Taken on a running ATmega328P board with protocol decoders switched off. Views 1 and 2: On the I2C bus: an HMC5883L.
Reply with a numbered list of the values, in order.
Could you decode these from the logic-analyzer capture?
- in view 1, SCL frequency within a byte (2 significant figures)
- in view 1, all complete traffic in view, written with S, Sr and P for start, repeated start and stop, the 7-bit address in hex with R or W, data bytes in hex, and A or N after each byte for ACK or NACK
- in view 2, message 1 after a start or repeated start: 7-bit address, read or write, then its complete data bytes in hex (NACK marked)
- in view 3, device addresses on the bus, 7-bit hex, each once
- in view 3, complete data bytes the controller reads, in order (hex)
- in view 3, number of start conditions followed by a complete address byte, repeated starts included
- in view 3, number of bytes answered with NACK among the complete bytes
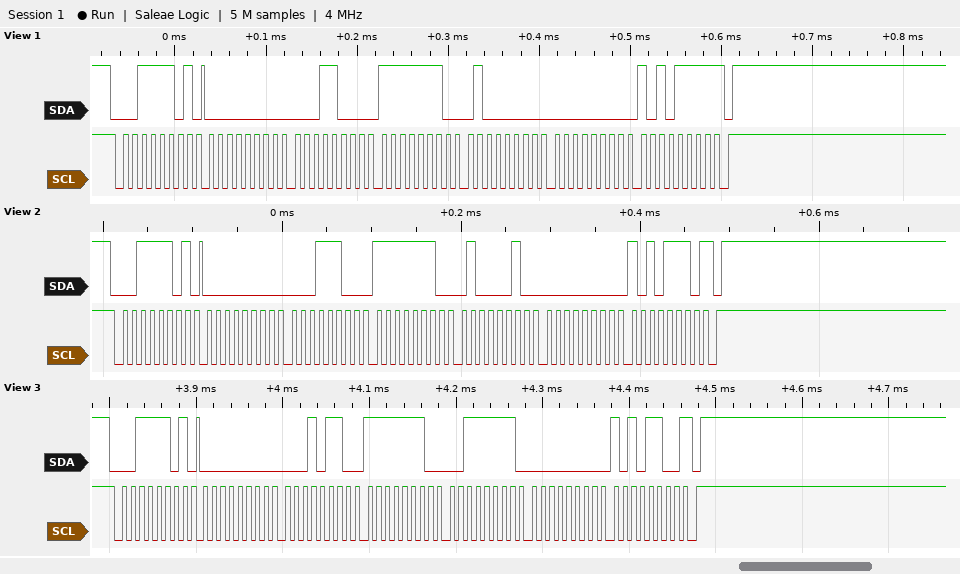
1. 100 kHz
2. S 1ER A 00 A 18 A FE A 40 A 00 A AF N P
3. 0x1E read: 00 1C FE 42 00 AE NACK
4. 0x1E
5. 00 16 FE 3F 00 AC
6. 1
7. 1
